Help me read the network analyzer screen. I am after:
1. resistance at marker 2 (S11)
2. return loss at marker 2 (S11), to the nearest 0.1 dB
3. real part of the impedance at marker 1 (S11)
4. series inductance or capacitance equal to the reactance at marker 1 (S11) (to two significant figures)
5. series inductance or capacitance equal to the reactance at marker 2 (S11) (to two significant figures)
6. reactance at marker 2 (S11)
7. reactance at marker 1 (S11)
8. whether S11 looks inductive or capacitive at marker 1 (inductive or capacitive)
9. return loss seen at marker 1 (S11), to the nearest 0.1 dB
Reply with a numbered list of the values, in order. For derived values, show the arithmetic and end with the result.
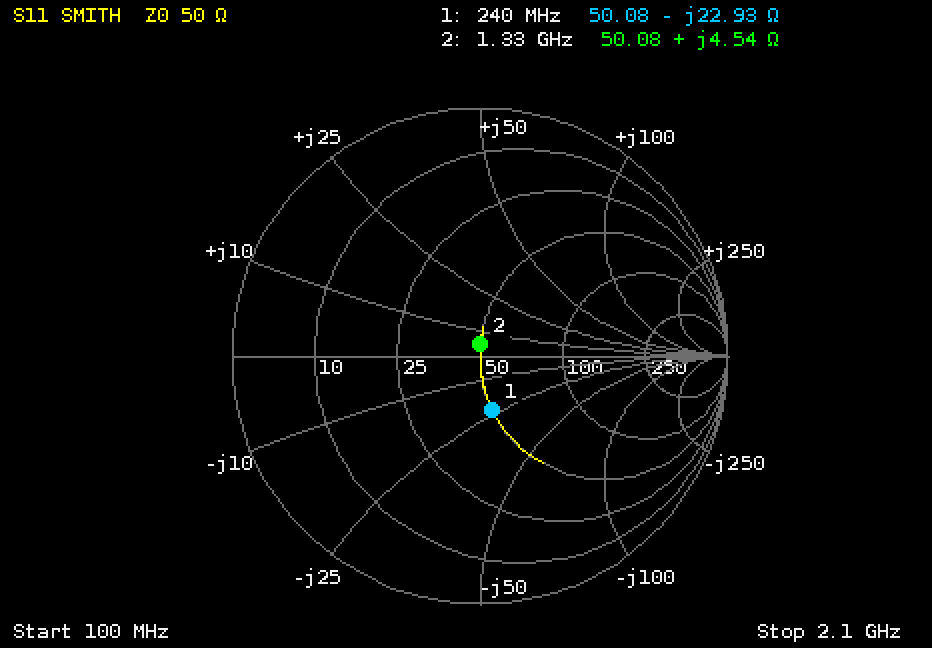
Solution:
1. 50.08 Ω
2. 26.9 dB
3. 50.08 Ω
4. C = 1/(2π × 240 MHz × 22.93 Ω) ≈ 29 pF
5. L = 4.54 Ω/(2π × 1.33 GHz) ≈ 543 pH, so 540 pH to two significant figures
6. +4.54 Ω
7. -22.93 Ω
8. capacitive
9. 13.0 dB
